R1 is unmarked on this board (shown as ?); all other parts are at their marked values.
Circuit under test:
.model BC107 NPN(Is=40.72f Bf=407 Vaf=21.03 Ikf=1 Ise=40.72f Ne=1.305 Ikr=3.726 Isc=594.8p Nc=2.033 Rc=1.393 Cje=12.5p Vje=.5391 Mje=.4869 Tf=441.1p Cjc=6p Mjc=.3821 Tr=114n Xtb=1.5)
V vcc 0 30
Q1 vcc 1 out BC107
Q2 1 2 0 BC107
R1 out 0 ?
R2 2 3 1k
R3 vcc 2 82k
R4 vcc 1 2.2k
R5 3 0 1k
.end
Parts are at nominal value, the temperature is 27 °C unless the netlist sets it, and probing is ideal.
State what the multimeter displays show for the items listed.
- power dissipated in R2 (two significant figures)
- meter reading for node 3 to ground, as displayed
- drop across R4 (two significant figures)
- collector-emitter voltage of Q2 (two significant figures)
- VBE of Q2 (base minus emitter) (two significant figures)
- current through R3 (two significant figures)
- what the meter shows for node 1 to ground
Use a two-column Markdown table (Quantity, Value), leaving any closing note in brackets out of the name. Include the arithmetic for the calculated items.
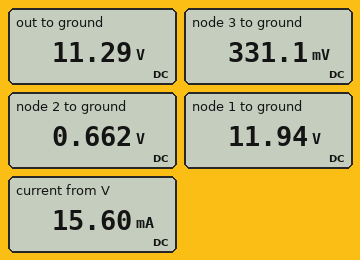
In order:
| Quantity | Value |
|---|---|
| power dissipated in R2 | (662 mV - 331.1 mV)^2 / 1 kΩ = 110 µW |
| meter reading for node 3 to ground, as displayed | 331.1 mV |
| drop across R4 | 30 V - 11.94 V = 18 V |
| collector-emitter voltage of Q2 | 11.94 V = 12 V |
| VBE of Q2 (base minus emitter) | 662 mV = 660 mV |
| current through R3 | (30 V - 662 mV) / 82 kΩ = 360 µA |
| what the meter shows for node 1 to ground | 11.94 V |
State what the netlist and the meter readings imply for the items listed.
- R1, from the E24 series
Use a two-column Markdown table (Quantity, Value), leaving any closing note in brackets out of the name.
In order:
| Quantity | Value |
|---|---|
| R1, from the E24 series | 1.6 kΩ |
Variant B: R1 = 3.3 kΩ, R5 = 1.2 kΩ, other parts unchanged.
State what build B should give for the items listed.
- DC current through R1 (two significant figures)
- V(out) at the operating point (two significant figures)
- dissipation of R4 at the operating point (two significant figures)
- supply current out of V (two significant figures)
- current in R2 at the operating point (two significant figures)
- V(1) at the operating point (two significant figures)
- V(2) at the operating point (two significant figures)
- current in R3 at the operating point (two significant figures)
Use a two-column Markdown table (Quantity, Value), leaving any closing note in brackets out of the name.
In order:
| Quantity | Value |
|---|---|
| DC current through R1 | 950 µA |
| V(out) at the operating point | 3.1 V |
| dissipation of R4 at the operating point | 310 mW |
| supply current out of V | 13 mA |
| current in R2 at the operating point | 310 µA |
| V(1) at the operating point | 3.7 V |
| V(2) at the operating point | 680 mV |
| current in R3 at the operating point | 360 µA |
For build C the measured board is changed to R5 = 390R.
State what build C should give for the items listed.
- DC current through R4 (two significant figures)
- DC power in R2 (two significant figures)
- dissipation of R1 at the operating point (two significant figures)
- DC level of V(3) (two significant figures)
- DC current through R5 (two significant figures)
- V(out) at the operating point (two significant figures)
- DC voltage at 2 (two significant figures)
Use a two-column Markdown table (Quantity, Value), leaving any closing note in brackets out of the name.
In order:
| Quantity | Value |
|---|---|
| DC current through R4 | 100 µA |
| DC power in R2 | 130 µW |
| dissipation of R1 at the operating point | 530 mW |
| DC level of V(3) | 140 mV |
| DC current through R5 | 360 µA |
| V(out) at the operating point | 29 V |
| DC voltage at 2 | 500 mV |
